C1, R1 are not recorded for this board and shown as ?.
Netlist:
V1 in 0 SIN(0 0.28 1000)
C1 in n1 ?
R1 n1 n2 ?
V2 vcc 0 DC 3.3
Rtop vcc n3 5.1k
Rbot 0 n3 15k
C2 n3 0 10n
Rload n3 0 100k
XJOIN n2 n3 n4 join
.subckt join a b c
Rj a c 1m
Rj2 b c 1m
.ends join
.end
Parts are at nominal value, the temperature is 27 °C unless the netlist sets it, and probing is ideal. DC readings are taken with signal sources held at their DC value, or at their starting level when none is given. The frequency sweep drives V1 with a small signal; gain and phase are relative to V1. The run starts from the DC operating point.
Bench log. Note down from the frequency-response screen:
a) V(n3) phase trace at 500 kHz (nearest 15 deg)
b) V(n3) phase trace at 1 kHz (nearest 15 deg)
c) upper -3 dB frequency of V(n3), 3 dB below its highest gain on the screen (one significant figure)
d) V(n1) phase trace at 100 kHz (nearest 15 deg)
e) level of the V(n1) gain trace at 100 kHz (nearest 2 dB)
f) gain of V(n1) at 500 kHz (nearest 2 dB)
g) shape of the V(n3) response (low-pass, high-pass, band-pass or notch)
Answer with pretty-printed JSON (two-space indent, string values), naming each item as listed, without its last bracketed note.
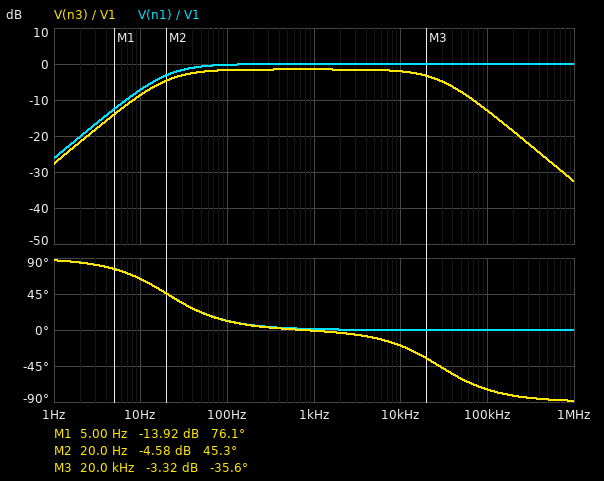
{
  "V(n3) phase trace at 500 kHz": "-90 deg",
  "V(n3) phase trace at 1 kHz": "0 deg",
  "upper -3 dB frequency of V(n3), 3 dB below its highest gain on the screen": "30 kHz",
  "V(n1) phase trace at 100 kHz": "0 deg",
  "level of the V(n1) gain trace at 100 kHz": "0 dB",
  "gain of V(n1) at 500 kHz": "0 dB",
  "shape of the V(n3) response": "band-pass"
}
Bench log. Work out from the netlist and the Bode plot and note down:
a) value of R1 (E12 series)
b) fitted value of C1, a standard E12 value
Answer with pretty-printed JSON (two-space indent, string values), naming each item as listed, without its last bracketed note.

{
  "value of R1": "680 Ω",
  "fitted value of C1, a standard E12 value": "1.8 µF"
}
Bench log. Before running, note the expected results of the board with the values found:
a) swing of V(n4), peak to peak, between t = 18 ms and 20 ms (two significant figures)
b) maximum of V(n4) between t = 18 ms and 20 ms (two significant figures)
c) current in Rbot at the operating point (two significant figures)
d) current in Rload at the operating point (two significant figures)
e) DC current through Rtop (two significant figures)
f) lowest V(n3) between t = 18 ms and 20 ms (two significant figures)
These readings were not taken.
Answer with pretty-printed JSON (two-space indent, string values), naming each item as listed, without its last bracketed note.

{
  "swing of V(n4), peak to peak, between t = 18 ms and 20 ms": "470 mV",
  "maximum of V(n4) between t = 18 ms and 20 ms": "2.6 V",
  "current in Rbot at the operating point": "160 µA",
  "current in Rload at the operating point": "24 µA",
  "DC current through Rtop": "180 µA",
  "lowest V(n3) between t = 18 ms and 20 ms": "2.1 V"
}
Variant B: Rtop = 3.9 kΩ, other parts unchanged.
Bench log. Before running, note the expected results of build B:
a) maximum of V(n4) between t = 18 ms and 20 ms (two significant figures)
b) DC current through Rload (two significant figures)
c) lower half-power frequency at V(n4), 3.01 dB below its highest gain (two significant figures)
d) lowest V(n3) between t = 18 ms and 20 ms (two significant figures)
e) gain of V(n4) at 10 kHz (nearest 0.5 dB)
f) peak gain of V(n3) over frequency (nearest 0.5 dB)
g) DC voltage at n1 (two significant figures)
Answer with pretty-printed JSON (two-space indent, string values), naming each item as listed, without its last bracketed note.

{
  "maximum of V(n4) between t = 18 ms and 20 ms": "2.8 V",
  "DC current through Rload": "25 µA",
  "lower half-power frequency at V(n4), 3.01 dB below its highest gain": "24 Hz",
  "lowest V(n3) between t = 18 ms and 20 ms": "2.3 V",
  "gain of V(n4) at 10 kHz": "-2.5 dB",
  "peak gain of V(n3) over frequency": "-2.0 dB",
  "DC voltage at n1": "2.5 V"
}
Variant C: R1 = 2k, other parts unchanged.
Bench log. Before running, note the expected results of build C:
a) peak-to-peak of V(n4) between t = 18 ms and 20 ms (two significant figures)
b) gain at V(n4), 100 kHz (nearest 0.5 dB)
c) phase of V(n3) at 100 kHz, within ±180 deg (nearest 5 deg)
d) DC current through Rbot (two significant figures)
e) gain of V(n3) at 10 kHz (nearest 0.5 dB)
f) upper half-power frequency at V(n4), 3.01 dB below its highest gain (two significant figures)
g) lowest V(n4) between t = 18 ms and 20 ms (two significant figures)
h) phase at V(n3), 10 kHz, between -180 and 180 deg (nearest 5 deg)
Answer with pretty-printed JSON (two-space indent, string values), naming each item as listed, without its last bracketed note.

{
  "peak-to-peak of V(n4) between t = 18 ms and 20 ms": "360 mV",
  "gain at V(n4), 100 kHz": "-22.0 dB",
  "phase of V(n3) at 100 kHz, within ±180 deg": "-85 deg",
  "DC current through Rbot": "160 µA",
  "gain of V(n3) at 10 kHz": "-6.0 dB",
  "upper half-power frequency at V(n4), 3.01 dB below its highest gain": "12 kHz",
  "lowest V(n4) between t = 18 ms and 20 ms": "2.2 V",
  "phase at V(n3), 10 kHz, between -180 and 180 deg": "-40 deg"
}
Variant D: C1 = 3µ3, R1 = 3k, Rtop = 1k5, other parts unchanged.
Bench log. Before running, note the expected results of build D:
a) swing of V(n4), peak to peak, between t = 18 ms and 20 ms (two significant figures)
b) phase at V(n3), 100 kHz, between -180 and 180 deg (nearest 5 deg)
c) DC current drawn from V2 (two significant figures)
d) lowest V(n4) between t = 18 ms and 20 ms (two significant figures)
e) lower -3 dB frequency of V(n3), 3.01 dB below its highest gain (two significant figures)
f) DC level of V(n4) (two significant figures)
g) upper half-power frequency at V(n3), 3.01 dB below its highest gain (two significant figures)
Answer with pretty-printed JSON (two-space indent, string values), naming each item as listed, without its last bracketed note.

{
  "swing of V(n4), peak to peak, between t = 18 ms and 20 ms": "170 mV",
  "phase at V(n3), 100 kHz, between -180 and 180 deg": "-80 deg",
  "DC current drawn from V2": "230 µA",
  "lowest V(n4) between t = 18 ms and 20 ms": "2.9 V",
  "lower -3 dB frequency of V(n3), 3.01 dB below its highest gain": "11 Hz",
  "DC level of V(n4)": "3.0 V",
  "upper half-power frequency at V(n3), 3.01 dB below its highest gain": "17 kHz"
}
